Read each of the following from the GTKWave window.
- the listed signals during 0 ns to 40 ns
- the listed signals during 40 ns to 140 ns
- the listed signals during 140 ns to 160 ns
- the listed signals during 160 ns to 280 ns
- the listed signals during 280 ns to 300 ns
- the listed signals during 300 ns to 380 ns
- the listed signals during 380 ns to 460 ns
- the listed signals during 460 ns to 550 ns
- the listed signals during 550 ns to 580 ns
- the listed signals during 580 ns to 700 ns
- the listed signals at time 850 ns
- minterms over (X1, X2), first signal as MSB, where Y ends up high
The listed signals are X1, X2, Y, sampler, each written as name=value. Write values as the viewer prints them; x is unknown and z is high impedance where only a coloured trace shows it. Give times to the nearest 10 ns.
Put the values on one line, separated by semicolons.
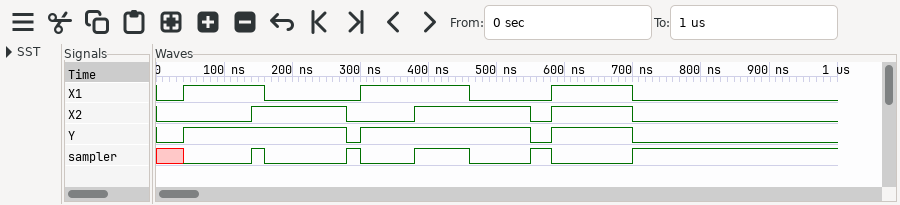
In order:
X1=0, X2=0, Y=0, sampler=x; X1=1, X2=0, Y=1, sampler=0; X1=1, X2=1, Y=1, sampler=1; X1=0, X2=1, Y=1, sampler=0; X1=0, X2=0, Y=0, sampler=1; X1=1, X2=0, Y=1, sampler=0; X1=1, X2=1, Y=1, sampler=1; X1=0, X2=1, Y=1, sampler=0; X1=0, X2=0, Y=0, sampler=1; X1=1, X2=1, Y=1, sampler=0; X1=0, X2=0, Y=0, sampler=1; 1, 2, 3
